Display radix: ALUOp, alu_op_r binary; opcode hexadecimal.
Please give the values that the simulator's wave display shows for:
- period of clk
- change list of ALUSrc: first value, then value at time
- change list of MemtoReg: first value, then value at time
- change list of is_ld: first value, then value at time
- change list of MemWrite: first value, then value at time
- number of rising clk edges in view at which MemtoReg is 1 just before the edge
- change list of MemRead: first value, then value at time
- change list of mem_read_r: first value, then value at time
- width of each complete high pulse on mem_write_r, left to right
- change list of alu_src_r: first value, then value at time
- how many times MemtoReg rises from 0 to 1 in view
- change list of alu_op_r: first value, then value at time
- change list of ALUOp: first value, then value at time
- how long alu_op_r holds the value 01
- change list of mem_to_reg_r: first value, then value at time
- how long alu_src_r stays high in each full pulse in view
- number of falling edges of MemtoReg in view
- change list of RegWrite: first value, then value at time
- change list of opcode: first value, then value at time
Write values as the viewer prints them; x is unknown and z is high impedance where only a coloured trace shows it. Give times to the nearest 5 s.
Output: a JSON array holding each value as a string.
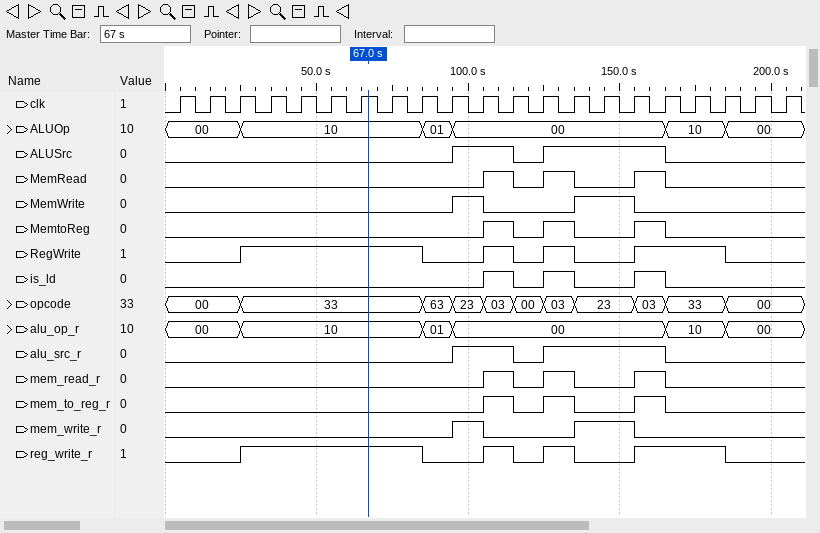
["10 s", "0, 1 at 95 s, 0 at 115 s, 1 at 125 s, 0 at 165 s", "0, 1 at 105 s, 0 at 115 s, 1 at 125 s, 0 at 135 s, 1 at 155 s, 0 at 165 s", "0, 1 at 105 s, 0 at 115 s, 1 at 125 s, 0 at 135 s, 1 at 155 s, 0 at 165 s", "0, 1 at 95 s, 0 at 105 s, 1 at 135 s, 0 at 155 s", "3", "0, 1 at 105 s, 0 at 115 s, 1 at 125 s, 0 at 135 s, 1 at 155 s, 0 at 165 s", "0, 1 at 105 s, 0 at 115 s, 1 at 125 s, 0 at 135 s, 1 at 155 s, 0 at 165 s", "10 s, 20 s", "0, 1 at 95 s, 0 at 115 s, 1 at 125 s, 0 at 165 s", "3", "00, 10 at 25 s, 01 at 85 s, 00 at 95 s, 10 at 165 s, 00 at 185 s", "00, 10 at 25 s, 01 at 85 s, 00 at 95 s, 10 at 165 s, 00 at 185 s", "10 s", "0, 1 at 105 s, 0 at 115 s, 1 at 125 s, 0 at 135 s, 1 at 155 s, 0 at 165 s", "20 s, 40 s", "3", "0, 1 at 25 s, 0 at 85 s, 1 at 105 s, 0 at 115 s, 1 at 125 s, 0 at 135 s, 1 at 155 s, 0 at 185 s", "00, 33 at 25 s, 63 at 85 s, 23 at 95 s, 03 at 105 s, 00 at 115 s, 03 at 125 s, 23 at 135 s, 03 at 155 s, 33 at 165 s, 00 at 185 s"]
